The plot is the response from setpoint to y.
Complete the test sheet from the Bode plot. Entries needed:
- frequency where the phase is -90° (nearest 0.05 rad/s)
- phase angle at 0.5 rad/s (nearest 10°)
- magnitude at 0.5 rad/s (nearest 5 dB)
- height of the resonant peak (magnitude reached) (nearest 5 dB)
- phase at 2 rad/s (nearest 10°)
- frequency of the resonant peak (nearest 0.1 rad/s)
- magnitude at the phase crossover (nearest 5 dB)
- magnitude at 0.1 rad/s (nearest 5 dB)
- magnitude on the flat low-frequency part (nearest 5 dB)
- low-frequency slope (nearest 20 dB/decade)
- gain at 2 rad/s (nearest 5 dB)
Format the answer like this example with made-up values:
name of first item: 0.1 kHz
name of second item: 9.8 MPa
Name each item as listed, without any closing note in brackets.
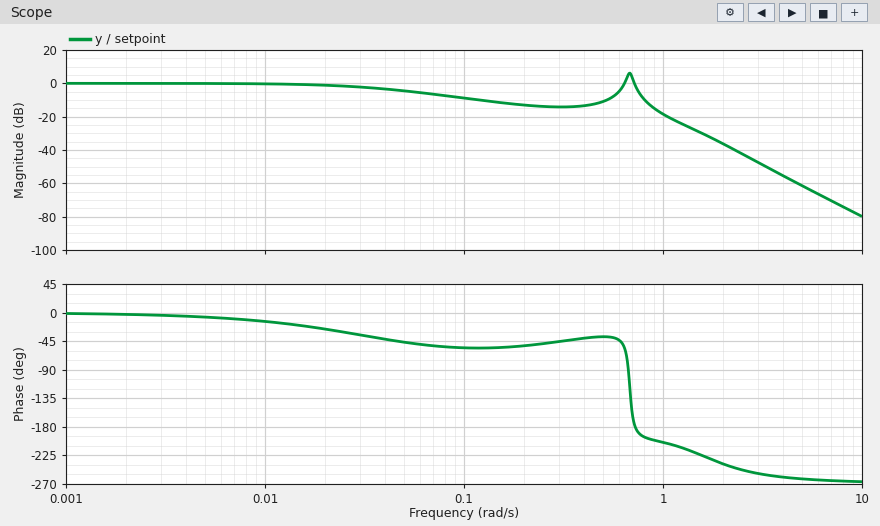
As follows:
frequency where the phase is -90°: 0.65 rad/s
phase angle at 0.5 rad/s: -40°
magnitude at 0.5 rad/s: -10 dB
height of the resonant peak (magnitude reached): 5 dB
phase at 2 rad/s: -240°
frequency of the resonant peak: 0.7 rad/s
magnitude at the phase crossover: 0 dB
magnitude at 0.1 rad/s: -10 dB
magnitude on the flat low-frequency part: 0 dB
low-frequency slope: 0 dB/decade
gain at 2 rad/s: -35 dB
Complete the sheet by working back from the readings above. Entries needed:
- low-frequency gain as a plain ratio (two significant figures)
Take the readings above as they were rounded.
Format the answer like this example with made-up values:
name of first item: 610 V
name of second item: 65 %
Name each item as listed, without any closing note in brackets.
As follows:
low-frequency gain as a plain ratio: 1.0
